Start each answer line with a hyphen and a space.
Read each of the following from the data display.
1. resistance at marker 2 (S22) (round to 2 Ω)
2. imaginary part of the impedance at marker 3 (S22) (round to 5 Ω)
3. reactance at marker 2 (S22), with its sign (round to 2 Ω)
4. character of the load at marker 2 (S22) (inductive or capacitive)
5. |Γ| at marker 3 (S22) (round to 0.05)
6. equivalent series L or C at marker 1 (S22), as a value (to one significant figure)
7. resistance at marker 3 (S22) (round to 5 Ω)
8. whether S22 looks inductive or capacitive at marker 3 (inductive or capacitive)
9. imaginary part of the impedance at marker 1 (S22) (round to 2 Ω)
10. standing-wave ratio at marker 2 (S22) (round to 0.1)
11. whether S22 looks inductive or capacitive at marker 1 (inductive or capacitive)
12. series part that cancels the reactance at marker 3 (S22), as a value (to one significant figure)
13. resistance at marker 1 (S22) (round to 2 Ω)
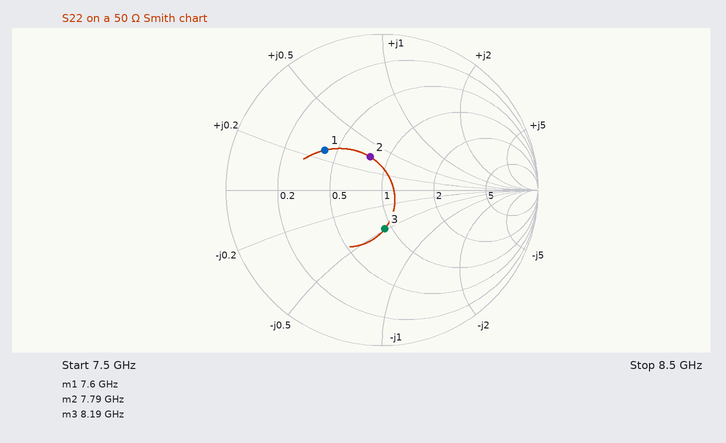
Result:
- 40 Ω
- -25 Ω
- +18 Ω
- inductive
- 0.25
- 300 pH
- 45 Ω
- capacitive
- +14 Ω
- 1.6
- inductive
- 500 pH
- 20 Ω
